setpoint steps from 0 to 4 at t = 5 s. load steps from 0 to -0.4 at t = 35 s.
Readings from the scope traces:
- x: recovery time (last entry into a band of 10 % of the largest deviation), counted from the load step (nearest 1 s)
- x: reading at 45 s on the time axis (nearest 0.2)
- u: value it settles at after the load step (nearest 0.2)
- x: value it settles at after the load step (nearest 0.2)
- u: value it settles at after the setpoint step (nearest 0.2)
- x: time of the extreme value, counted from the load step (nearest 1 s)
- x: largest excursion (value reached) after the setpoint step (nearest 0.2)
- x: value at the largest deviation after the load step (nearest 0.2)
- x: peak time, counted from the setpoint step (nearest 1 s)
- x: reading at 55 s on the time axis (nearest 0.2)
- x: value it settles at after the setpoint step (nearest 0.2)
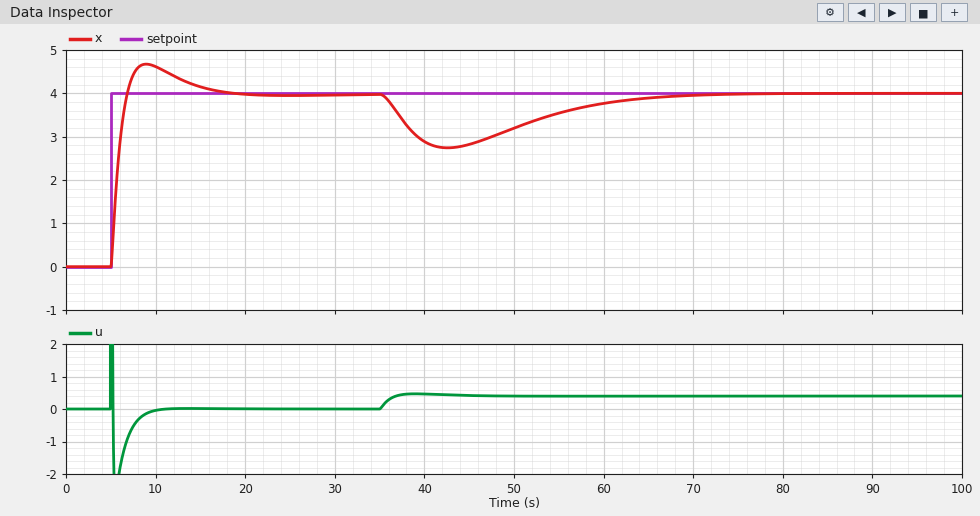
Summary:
29 s
2.8
0.4
4.0
0.0
8 s
4.6
2.8
4 s
3.6
4.0
